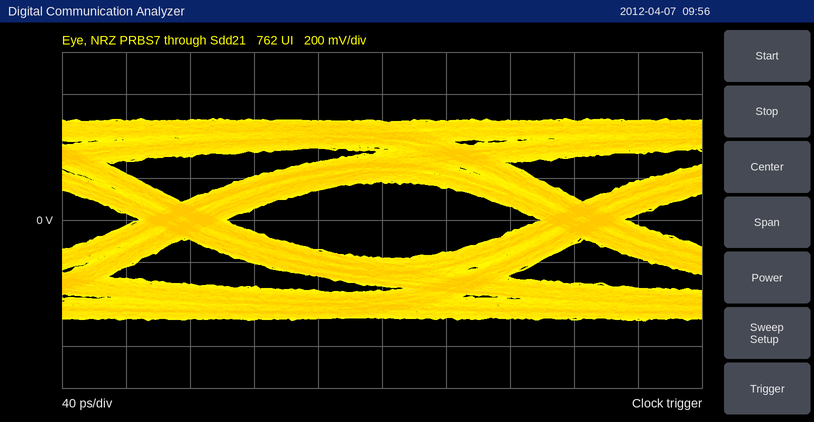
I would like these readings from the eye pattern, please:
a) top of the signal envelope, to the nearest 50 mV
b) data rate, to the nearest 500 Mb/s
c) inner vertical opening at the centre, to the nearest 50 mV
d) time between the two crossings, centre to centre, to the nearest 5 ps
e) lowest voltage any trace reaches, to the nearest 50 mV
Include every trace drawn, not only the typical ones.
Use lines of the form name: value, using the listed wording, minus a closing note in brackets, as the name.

top of the signal envelope, to the nearest 50 mV: 500 mV
data rate, to the nearest 500 Mb/s: 4.0 Gb/s
inner vertical opening at the centre, to the nearest 50 mV: 350 mV
time between the two crossings, centre to centre, to the nearest 5 ps: 250 ps
lowest voltage any trace reaches, to the nearest 50 mV: -500 mV
